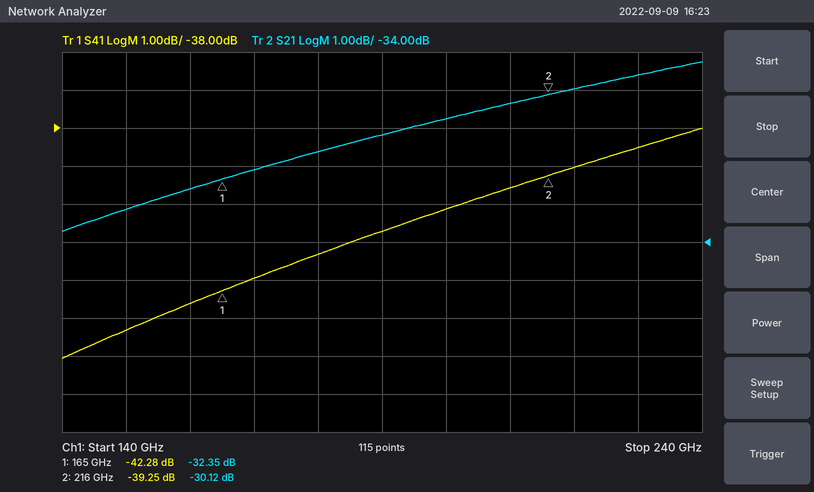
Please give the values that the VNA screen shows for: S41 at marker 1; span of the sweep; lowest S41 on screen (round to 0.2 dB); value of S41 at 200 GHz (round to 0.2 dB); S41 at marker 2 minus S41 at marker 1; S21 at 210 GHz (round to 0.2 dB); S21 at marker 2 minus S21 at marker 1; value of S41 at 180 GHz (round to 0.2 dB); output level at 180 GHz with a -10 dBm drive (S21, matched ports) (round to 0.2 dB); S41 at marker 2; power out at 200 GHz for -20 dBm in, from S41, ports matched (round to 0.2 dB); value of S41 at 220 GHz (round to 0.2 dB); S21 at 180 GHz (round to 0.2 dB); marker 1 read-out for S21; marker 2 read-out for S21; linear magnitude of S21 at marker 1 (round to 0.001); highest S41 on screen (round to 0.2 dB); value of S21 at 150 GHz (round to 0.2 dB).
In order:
-42.28 dB
100 GHz
-44.0 dB
-40.2 dB
3.03 dB
-30.4 dB
2.23 dB
-41.4 dB
-41.6 dBm
-39.25 dB
-60.2 dBm
-39.0 dB
-31.6 dB
-32.35 dB
-30.12 dB
0.024
-38.0 dB
-33.2 dB
